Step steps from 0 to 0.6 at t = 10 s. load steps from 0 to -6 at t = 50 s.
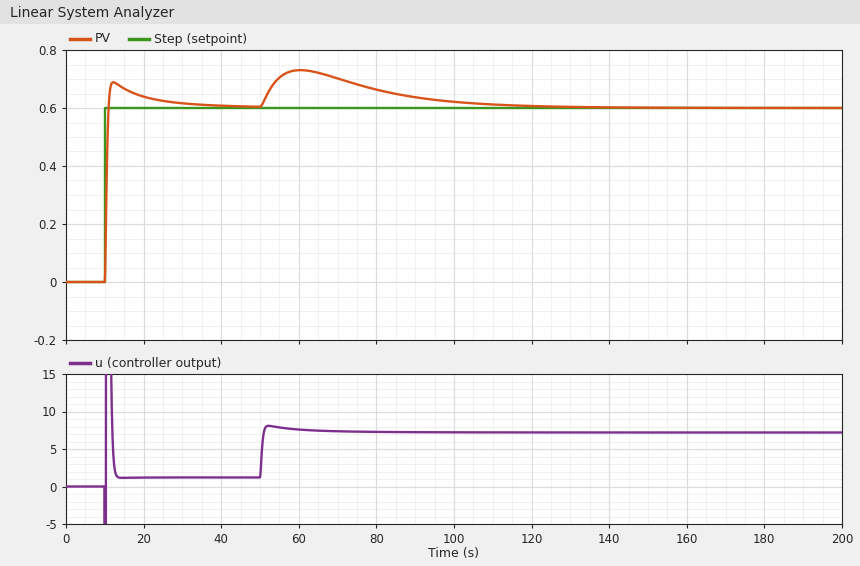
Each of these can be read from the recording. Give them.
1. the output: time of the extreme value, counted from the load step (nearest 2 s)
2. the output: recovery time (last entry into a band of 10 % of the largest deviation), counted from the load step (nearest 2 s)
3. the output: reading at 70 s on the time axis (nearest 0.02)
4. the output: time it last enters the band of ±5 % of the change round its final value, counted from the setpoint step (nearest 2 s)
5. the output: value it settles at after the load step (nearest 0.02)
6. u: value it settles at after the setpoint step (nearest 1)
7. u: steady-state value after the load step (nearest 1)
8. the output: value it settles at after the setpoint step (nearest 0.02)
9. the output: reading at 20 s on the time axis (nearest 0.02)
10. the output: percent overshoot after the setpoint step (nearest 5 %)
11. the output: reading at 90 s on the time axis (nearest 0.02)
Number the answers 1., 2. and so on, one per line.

1. 10 s
2. 60 s
3. 0.70
4. 12 s
5. 0.60
6. 1
7. 7
8. 0.60
9. 0.64
10. 15 %
11. 0.64
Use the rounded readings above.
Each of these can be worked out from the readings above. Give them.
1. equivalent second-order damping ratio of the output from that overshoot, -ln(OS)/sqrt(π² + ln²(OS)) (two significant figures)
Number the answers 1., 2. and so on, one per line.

1. 0.52
